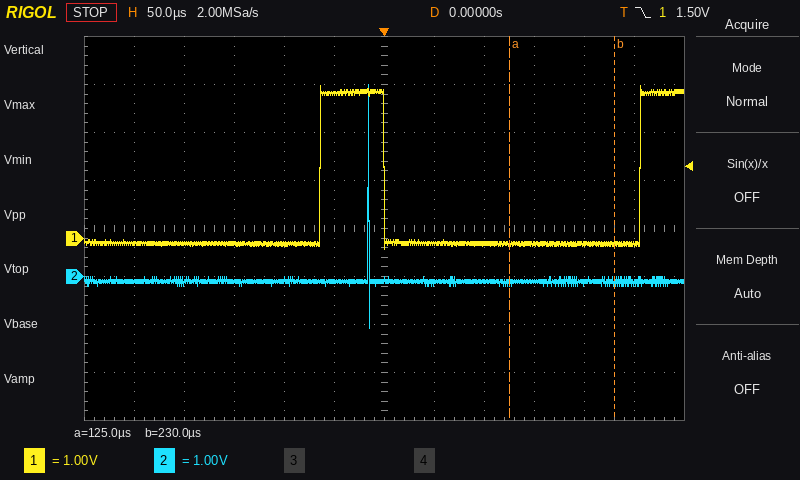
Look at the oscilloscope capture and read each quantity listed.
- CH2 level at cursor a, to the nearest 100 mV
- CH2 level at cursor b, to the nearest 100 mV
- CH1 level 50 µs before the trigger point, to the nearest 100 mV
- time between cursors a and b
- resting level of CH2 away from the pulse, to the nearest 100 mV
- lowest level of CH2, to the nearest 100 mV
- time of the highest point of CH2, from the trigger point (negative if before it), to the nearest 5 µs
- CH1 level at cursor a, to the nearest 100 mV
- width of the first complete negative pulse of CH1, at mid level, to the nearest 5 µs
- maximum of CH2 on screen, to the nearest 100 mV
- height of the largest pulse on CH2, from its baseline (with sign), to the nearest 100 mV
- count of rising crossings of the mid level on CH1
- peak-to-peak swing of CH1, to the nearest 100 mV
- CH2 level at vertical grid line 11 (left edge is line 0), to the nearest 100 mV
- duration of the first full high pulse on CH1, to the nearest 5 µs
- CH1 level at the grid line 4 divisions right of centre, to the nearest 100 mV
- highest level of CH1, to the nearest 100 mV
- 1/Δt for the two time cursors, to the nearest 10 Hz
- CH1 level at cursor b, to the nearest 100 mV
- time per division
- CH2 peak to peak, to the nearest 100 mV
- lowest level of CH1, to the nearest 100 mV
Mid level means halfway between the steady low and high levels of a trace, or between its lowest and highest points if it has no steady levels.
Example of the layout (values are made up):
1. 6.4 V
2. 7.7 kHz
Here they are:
1. -100 mV
2. -100 mV
3. 3.0 V
4. 105 µs
5. -100 mV
6. -1.1 V
7. -15 µs
8. -100 mV
9. 255 µs
10. 4.0 V
11. +4.1 V
12. 2
13. 3.4 V
14. -100 mV
15. 65 µs
16. -100 mV
17. 3.2 V
18. 9.52 kHz
19. -100 mV
20. 50 µs
21. 5.1 V
22. -200 mV
